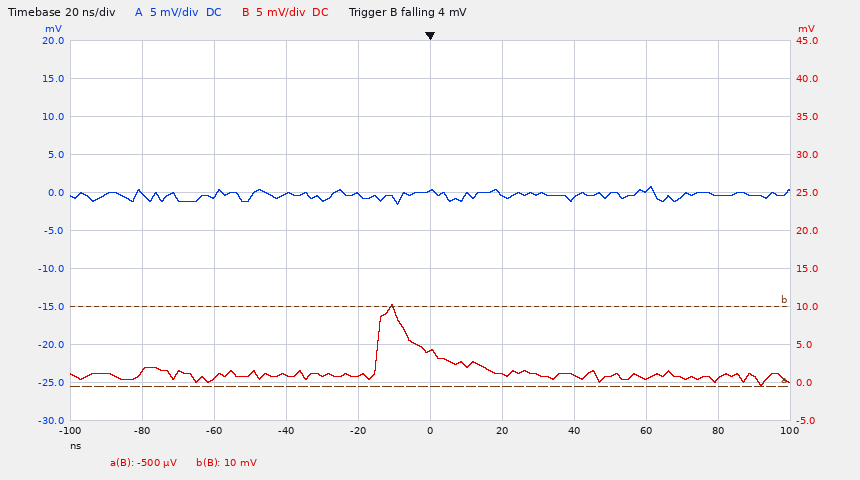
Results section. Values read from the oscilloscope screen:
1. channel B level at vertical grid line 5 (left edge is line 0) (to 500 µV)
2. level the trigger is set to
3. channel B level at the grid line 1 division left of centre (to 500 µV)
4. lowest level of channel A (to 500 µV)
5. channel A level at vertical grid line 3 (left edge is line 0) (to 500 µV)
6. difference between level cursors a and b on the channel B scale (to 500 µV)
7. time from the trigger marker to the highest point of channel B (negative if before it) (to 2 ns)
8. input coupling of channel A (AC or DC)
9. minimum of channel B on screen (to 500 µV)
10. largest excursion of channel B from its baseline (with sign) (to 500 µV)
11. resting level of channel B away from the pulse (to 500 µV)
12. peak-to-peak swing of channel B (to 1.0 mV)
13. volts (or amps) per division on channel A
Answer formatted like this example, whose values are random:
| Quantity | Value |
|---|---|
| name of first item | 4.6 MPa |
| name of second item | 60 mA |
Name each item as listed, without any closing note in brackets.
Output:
| Quantity | Value |
|---|---|
| channel B level at vertical grid line 5 (left edge is line 0) | 4.0 mV |
| level the trigger is set to | 4 mV |
| channel B level at the grid line 1 division left of centre | 1.0 mV |
| lowest level of channel A | -1.5 mV |
| channel A level at vertical grid line 3 (left edge is line 0) | 0.0 mV |
| difference between level cursors a and b on the channel B scale | 10.5 mV |
| time from the trigger marker to the highest point of channel B (negative if before it) | -10 ns |
| input coupling of channel A | DC |
| minimum of channel B on screen | -500 µV |
| largest excursion of channel B from its baseline (with sign) | +9.5 mV |
| resting level of channel B away from the pulse | 1.0 mV |
| peak-to-peak swing of channel B | 11.0 mV |
| volts (or amps) per division on channel A | 5 mV |
